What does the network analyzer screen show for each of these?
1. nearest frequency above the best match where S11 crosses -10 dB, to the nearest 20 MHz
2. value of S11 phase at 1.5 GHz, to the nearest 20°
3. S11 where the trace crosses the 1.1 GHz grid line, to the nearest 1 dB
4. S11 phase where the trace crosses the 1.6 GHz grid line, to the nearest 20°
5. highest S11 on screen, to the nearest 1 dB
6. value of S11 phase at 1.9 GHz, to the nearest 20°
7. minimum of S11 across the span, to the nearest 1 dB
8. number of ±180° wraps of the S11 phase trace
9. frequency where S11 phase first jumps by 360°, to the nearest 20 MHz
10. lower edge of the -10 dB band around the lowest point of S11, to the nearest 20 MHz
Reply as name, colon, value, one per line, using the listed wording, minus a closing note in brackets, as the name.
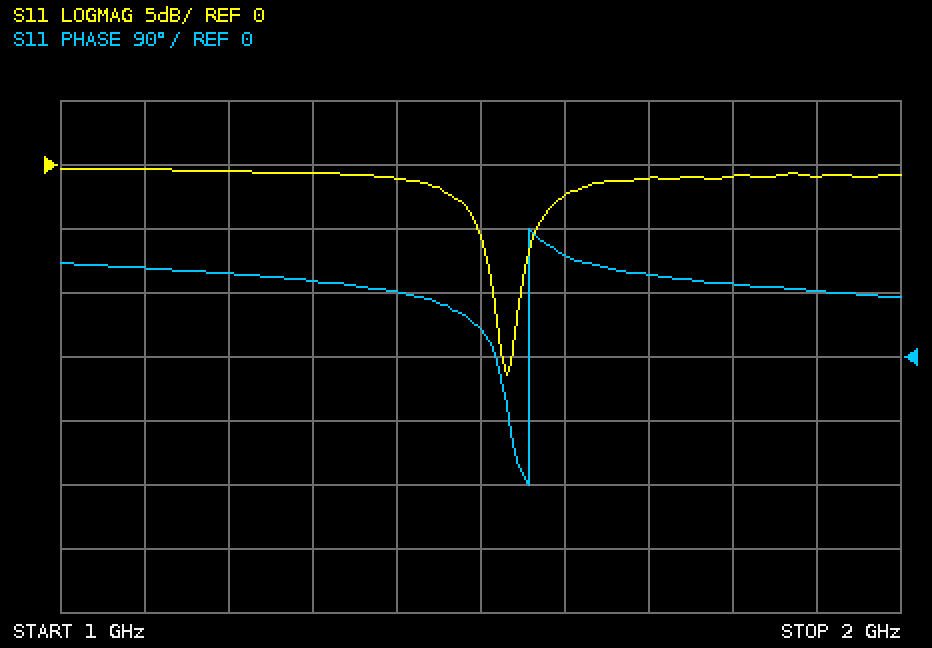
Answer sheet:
nearest frequency above the best match where S11 crosses -10 dB, to the nearest 20 MHz: 1.54 GHz
value of S11 phase at 1.5 GHz, to the nearest 20°: 40°
S11 where the trace crosses the 1.1 GHz grid line, to the nearest 1 dB: 0 dB
S11 phase where the trace crosses the 1.6 GHz grid line, to the nearest 20°: 140°
highest S11 on screen, to the nearest 1 dB: 0 dB
value of S11 phase at 1.9 GHz, to the nearest 20°: 100°
minimum of S11 across the span, to the nearest 1 dB: -16 dB
number of ±180° wraps of the S11 phase trace: 1
frequency where S11 phase first jumps by 360°, to the nearest 20 MHz: 1.56 GHz
lower edge of the -10 dB band around the lowest point of S11, to the nearest 20 MHz: 1.52 GHz
